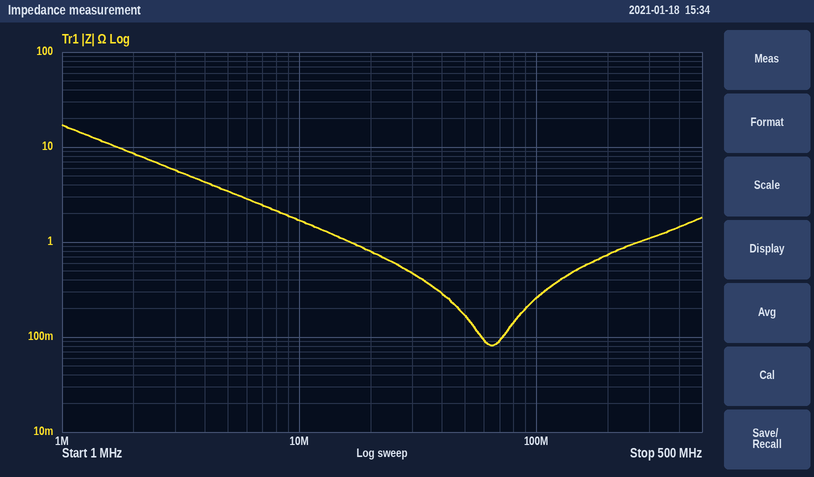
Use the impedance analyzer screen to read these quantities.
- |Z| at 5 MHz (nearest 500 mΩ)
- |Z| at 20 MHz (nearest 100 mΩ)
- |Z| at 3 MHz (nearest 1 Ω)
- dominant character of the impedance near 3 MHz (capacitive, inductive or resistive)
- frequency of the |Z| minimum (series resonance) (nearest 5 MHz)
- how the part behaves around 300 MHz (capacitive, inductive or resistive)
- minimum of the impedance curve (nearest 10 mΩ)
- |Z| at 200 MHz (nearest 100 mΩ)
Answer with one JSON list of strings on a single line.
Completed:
["3.5 Ω", "800 mΩ", "6 Ω", "capacitive", "65 MHz", "inductive", "80 mΩ", "700 mΩ"]
